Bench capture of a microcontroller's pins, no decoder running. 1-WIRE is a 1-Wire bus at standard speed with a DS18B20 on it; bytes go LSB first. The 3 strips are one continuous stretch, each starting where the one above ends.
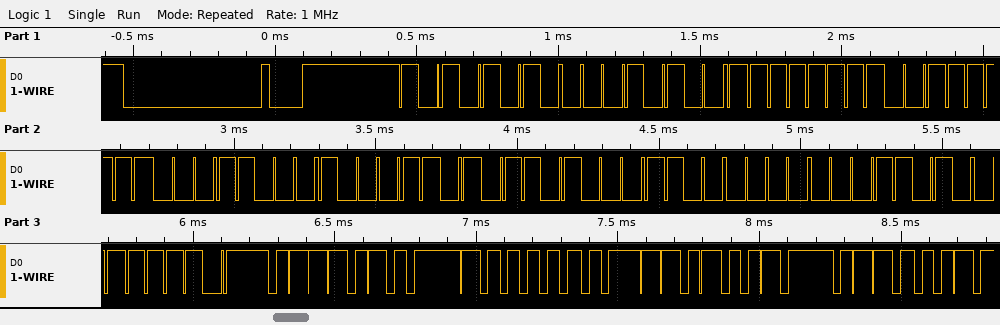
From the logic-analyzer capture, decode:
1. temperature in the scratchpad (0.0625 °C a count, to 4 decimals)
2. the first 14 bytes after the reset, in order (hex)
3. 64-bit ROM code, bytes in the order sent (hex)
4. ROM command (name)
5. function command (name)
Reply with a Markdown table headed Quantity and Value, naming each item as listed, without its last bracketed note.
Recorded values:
| Quantity | Value |
|---|---|
| temperature in the scratchpad | 18.8750 °C |
| the first 14 bytes after the reset, in order | 55 28 FF FC 18 B1 16 03 58 BE 2E 01 4B 46 |
| 64-bit ROM code, bytes in the order sent | 28 FF FC 18 B1 16 03 58 |
| ROM command | Match ROM |
| function command | Read Scratchpad |
